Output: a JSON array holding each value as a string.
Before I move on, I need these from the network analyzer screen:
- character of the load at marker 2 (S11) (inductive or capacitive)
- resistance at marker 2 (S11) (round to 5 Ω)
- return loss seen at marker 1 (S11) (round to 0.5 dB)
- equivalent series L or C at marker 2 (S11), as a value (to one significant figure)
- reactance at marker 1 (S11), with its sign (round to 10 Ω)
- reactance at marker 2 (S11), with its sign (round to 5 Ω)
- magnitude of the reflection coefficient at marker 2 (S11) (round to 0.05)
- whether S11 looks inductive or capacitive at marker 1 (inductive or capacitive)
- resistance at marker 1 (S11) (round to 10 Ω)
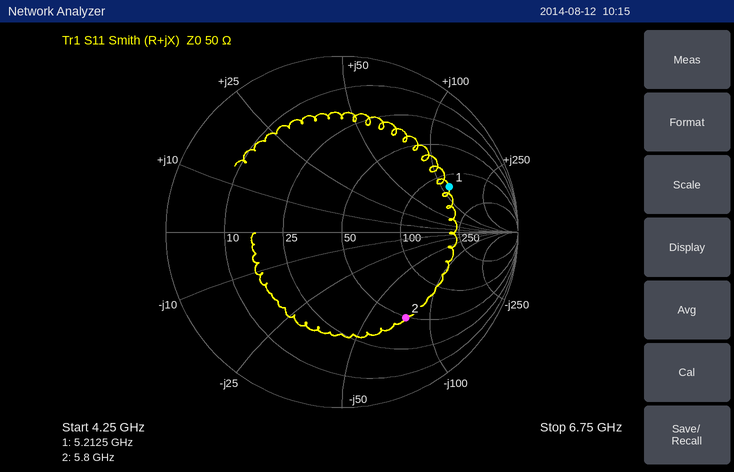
["capacitive", "50 Ω", "3.5 dB", "400 fF", "+120 Ω", "-75 Ω", "0.60", "inductive", "130 Ω"]
